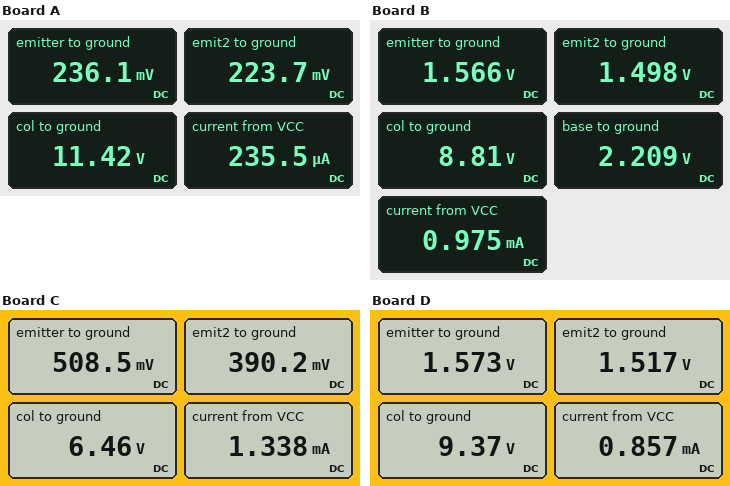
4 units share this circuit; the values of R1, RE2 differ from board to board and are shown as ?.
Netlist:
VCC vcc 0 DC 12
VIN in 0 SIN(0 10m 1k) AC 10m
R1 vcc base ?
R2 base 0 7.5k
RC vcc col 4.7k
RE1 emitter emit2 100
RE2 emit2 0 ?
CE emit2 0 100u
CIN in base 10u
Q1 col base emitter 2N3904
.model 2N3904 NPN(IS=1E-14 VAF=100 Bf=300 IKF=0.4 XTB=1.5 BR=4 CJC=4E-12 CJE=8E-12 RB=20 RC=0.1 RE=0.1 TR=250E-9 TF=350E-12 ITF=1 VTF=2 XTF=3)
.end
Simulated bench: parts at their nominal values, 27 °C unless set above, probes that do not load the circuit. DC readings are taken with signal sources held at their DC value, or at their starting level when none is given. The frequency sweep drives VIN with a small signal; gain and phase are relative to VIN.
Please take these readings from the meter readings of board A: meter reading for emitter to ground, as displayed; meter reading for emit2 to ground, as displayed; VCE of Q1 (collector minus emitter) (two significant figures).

236.1 mV
223.7 mV
11 V
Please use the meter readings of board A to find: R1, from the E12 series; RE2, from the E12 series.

100 kΩ
1.8 kΩ
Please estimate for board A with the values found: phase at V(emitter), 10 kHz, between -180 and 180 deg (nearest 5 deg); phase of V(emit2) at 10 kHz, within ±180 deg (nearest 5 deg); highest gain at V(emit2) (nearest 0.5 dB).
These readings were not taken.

0 deg
-90 deg
-4.5 dB
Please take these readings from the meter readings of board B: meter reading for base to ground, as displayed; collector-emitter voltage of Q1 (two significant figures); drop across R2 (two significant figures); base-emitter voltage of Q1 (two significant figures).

2.209 V
7.2 V
2.2 V
640 mV
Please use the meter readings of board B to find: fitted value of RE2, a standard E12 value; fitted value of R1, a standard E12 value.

2.2 kΩ
33 kΩ
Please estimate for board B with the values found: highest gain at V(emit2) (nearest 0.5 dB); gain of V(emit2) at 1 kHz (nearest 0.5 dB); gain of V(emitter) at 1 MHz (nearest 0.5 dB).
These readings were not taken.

-2.5 dB
-39.0 dB
-3.0 dB
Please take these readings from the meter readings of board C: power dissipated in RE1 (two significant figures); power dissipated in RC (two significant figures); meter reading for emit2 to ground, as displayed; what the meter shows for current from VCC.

140 µW
6.5 mW
390.2 mV
1.338 mA
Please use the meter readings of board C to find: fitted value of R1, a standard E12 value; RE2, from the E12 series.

68 kΩ
330 Ω
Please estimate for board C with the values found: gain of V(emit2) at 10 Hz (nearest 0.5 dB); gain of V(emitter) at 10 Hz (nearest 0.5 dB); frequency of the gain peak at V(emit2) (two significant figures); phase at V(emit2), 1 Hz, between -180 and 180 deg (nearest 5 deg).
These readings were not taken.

-4.5 dB
-1.0 dB
6.6 Hz
65 deg
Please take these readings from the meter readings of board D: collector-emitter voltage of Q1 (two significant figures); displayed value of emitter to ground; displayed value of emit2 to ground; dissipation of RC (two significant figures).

7.8 V
1.573 V
1.517 V
1.5 mW
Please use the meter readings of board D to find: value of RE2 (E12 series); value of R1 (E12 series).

2.7 kΩ
33 kΩ
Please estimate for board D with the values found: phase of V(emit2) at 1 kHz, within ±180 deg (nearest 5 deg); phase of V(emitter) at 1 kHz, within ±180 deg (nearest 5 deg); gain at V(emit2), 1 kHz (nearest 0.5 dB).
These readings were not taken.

-90 deg
0 deg
-39.5 dB
